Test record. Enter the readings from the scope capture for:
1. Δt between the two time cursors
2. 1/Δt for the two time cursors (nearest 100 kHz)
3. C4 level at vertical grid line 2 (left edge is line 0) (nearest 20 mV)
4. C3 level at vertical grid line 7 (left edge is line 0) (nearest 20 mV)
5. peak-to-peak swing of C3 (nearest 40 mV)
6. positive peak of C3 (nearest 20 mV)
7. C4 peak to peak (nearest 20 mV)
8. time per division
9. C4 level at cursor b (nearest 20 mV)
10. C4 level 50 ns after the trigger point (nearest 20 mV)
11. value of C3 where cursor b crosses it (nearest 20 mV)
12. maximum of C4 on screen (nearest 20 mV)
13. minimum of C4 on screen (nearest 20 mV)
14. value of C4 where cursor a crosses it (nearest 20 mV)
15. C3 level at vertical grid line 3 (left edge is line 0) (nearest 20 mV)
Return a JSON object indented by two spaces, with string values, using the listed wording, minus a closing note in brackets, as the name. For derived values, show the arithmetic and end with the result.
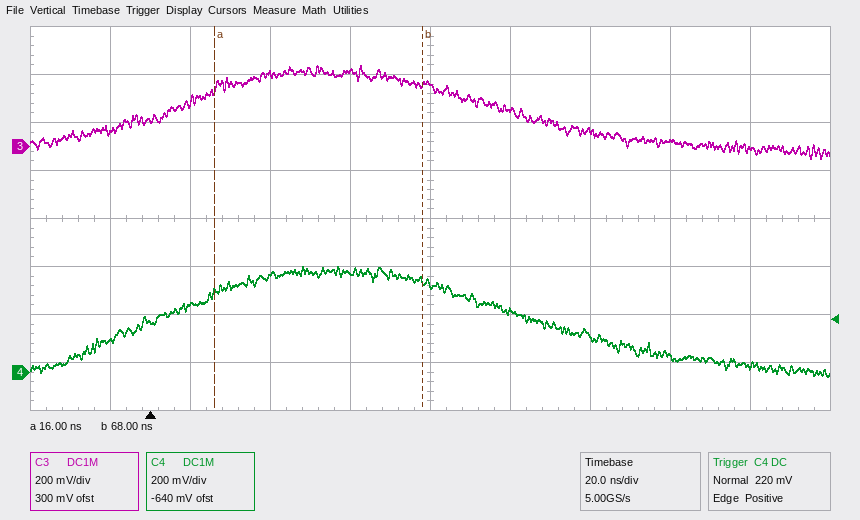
{
  "Δt between the two time cursors": "68 ns − (16 ns) = 52 ns",
  "1/Δt for the two time cursors": "1 / 52 ns ≈ 19.2 MHz",
  "C4 level at vertical grid line 2 (left edge is line 0)": "280 mV",
  "C3 level at vertical grid line 7 (left edge is line 0)": "60 mV",
  "peak-to-peak swing of C3": "400 mV",
  "positive peak of C3": "340 mV",
  "C4 peak to peak": "440 mV − (-20 mV) = 460 mV",
  "time per division": "20 ns",
  "C4 level at cursor b": "380 mV",
  "C4 level 50 ns after the trigger point": "420 mV",
  "value of C3 where cursor b crosses it": "260 mV",
  "maximum of C4 on screen": "440 mV",
  "minimum of C4 on screen": "-20 mV",
  "value of C4 where cursor a crosses it": "320 mV",
  "C3 level at vertical grid line 3 (left edge is line 0)": "300 mV"
}
